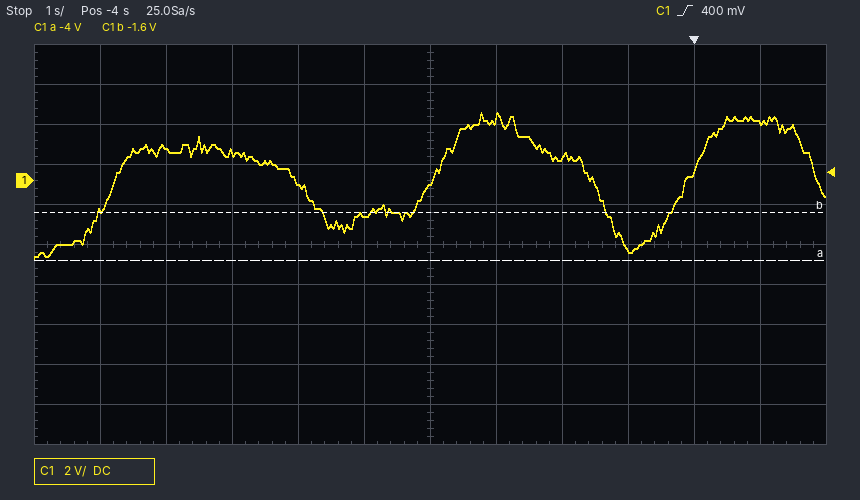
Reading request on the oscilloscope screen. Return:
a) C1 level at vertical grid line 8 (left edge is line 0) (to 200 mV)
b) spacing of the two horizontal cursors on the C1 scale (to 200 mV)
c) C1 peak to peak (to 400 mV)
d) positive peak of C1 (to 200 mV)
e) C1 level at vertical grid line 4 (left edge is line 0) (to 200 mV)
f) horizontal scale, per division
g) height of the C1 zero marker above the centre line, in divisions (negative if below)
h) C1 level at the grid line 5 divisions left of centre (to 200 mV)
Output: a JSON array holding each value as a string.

["1.2 V", "2.4 V", "7.2 V", "3.4 V", "-200 mV", "1 s", "+1.6 div", "-1.6 V"]
